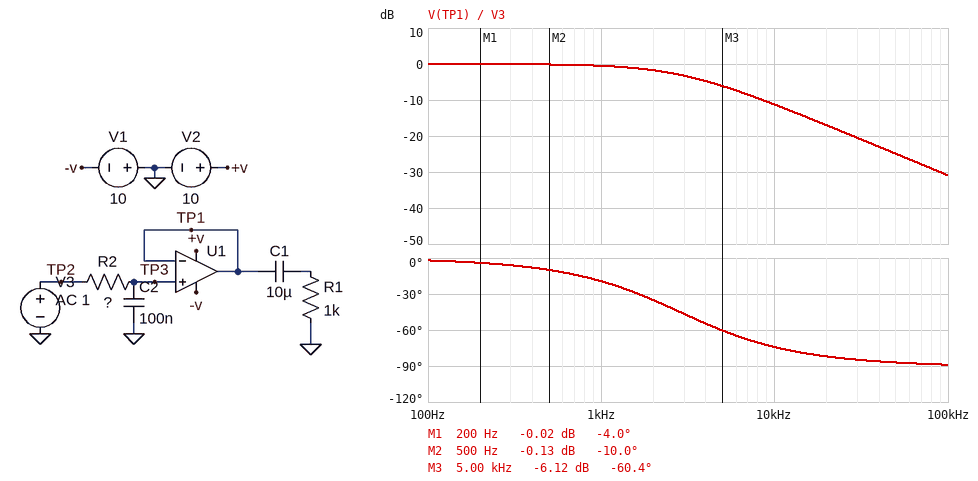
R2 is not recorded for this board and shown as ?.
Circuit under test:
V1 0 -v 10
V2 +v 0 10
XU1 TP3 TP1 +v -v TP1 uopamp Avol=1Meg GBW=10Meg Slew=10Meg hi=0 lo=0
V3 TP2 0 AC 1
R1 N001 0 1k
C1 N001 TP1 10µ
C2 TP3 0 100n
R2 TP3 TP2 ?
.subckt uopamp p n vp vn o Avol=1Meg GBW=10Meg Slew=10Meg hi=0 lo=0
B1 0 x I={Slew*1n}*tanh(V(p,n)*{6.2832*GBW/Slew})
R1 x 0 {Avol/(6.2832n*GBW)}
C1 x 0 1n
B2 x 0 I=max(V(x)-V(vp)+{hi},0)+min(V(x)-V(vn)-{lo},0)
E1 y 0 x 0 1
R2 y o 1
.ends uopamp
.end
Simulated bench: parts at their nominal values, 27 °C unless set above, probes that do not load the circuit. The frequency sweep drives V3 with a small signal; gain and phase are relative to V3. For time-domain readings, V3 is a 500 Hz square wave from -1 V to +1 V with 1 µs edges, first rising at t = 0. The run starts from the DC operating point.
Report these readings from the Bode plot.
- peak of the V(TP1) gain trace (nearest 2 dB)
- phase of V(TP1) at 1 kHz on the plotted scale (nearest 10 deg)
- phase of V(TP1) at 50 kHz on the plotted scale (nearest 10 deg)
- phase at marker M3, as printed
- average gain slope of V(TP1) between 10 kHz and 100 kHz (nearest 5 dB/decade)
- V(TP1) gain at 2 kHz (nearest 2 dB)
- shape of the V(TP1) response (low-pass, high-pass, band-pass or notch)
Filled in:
0 dB
-20 deg
-90 deg
-60.4 deg
-20 dB/decade
-2 dB
low-pass
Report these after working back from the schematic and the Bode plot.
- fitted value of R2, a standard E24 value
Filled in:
560 Ω
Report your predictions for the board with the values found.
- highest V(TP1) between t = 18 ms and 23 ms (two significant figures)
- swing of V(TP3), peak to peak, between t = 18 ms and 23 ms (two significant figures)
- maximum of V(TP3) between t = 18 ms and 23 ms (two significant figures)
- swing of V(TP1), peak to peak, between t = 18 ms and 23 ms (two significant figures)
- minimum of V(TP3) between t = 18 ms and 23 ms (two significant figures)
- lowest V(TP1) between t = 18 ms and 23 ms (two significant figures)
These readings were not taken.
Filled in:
1.0 V
2.0 V
1.0 V
2.0 V
-1.0 V
-1.0 V
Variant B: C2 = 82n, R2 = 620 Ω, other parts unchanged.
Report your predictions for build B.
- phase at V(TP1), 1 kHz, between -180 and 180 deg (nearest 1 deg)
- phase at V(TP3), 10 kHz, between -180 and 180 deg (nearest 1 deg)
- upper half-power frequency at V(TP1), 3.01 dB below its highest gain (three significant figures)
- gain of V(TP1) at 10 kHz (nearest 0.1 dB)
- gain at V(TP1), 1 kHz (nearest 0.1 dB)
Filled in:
-18 deg
-73 deg
3.13 kHz
-10.5 dB
-0.4 dB
